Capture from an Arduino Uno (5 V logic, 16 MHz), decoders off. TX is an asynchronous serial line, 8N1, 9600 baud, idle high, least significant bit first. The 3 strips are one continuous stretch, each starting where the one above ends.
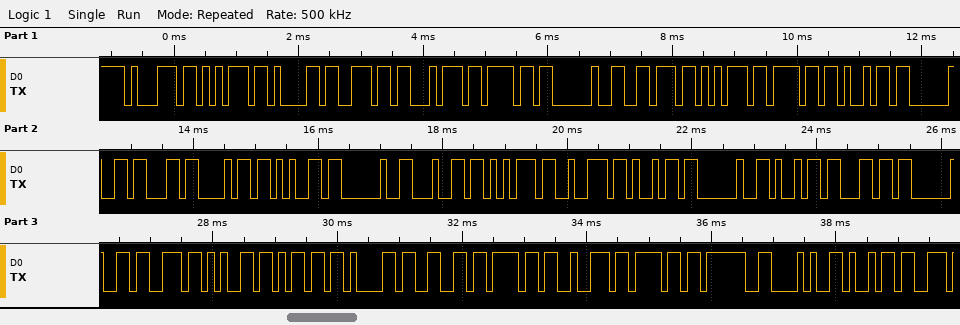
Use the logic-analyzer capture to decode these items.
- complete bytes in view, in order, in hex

71 75 61 6E 74 6F 20 76 75 6F 69 20 63 68 65 20 64 75 72 69 20 69 6C 20 73 65 6D 61 66 6F 72 6F 3F 28 69
